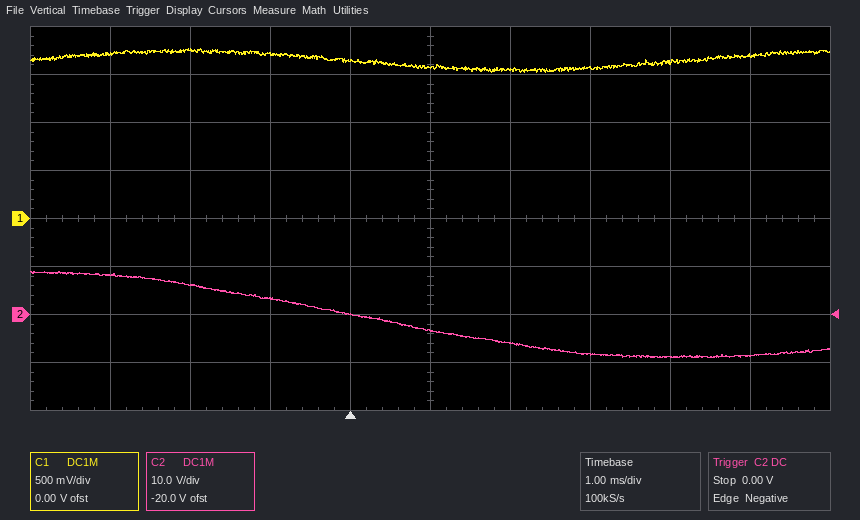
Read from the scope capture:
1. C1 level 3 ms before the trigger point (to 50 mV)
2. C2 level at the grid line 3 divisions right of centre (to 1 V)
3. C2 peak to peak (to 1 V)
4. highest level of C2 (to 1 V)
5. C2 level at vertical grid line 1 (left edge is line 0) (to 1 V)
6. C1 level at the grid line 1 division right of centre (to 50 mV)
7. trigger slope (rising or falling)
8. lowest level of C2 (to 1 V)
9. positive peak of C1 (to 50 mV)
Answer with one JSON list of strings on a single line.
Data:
["1.70 V", "-9 V", "18 V", "9 V", "8 V", "1.55 V", "falling", "-9 V", "1.75 V"]
